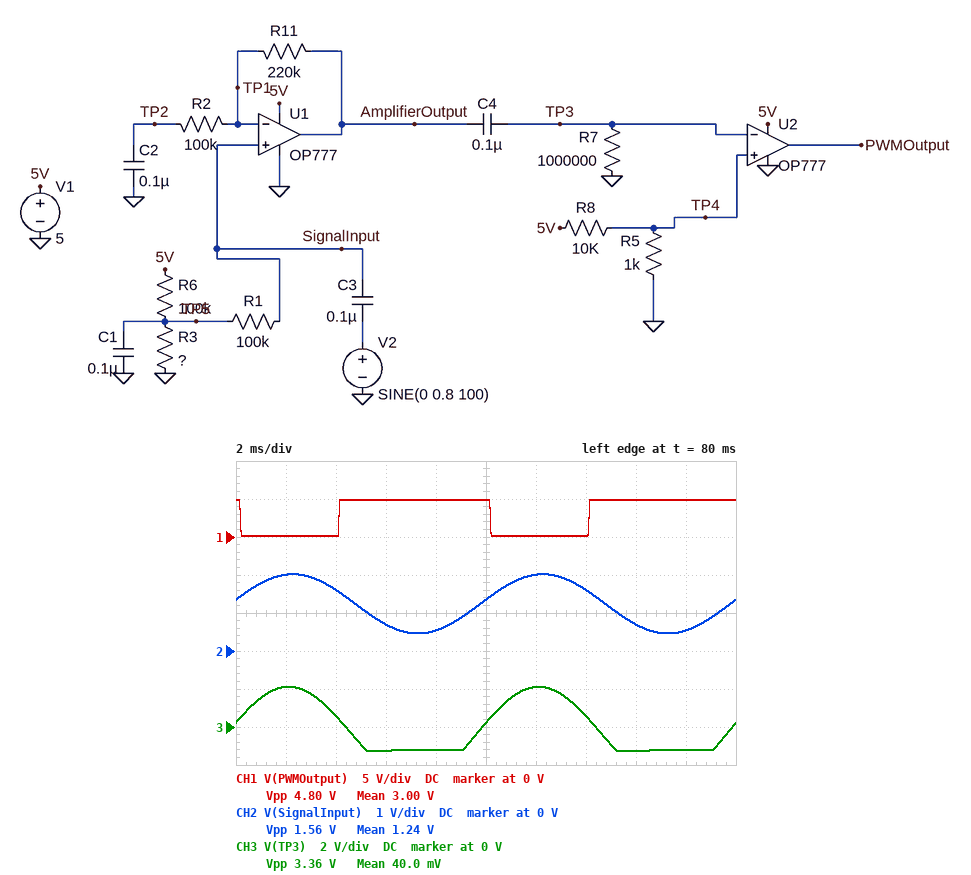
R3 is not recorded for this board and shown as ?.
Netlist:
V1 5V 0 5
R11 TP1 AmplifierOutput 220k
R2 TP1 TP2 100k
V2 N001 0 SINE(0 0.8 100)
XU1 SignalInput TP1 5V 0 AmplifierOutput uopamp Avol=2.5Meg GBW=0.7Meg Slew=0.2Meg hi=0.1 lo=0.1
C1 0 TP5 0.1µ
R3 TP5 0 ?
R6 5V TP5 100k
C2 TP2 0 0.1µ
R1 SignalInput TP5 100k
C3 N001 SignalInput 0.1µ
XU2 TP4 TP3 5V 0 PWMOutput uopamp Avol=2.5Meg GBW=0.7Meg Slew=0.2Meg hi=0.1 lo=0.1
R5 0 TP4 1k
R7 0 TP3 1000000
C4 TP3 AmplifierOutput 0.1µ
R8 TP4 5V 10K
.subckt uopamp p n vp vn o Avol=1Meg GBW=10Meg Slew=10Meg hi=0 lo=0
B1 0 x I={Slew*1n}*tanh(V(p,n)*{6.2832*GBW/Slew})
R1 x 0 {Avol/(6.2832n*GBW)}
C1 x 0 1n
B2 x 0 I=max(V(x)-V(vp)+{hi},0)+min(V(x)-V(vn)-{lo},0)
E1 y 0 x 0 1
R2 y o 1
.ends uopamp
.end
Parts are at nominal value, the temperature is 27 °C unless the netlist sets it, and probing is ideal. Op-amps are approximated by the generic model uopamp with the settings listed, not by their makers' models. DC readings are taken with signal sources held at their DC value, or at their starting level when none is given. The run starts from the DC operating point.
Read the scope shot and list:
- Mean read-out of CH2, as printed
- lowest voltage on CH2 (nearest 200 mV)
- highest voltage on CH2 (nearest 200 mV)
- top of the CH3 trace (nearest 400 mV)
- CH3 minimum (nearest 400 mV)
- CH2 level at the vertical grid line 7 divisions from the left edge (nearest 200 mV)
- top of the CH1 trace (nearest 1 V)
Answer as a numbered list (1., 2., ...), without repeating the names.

1. 1.24 V
2. 400 mV
3. 2.0 V
4. 2.0 V
5. -1.2 V
6. 1.6 V
7. 5 V
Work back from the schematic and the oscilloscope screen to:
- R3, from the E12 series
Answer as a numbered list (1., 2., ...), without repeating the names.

1. 33 kΩ
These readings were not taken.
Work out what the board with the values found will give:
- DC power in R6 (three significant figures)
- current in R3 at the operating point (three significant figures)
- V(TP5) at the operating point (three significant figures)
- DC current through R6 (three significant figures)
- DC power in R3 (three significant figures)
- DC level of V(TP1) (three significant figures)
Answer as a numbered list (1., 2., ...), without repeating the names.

1. 141 µW
2. 37.6 µA
3. 1.24 V
4. 37.6 µA
5. 46.6 µW
6. 1.24 V
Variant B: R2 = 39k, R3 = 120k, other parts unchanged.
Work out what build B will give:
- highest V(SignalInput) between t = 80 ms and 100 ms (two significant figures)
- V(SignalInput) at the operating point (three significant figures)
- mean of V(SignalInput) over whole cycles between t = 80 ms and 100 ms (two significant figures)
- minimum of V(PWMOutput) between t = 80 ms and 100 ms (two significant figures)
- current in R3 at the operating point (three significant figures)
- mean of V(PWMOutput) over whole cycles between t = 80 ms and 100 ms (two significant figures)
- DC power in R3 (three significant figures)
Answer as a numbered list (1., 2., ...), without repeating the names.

1. 3.5 V
2. 2.73 V
3. 2.7 V
4. 100 mV
5. 22.7 µA
6. 2.5 V
7. 62.0 µW
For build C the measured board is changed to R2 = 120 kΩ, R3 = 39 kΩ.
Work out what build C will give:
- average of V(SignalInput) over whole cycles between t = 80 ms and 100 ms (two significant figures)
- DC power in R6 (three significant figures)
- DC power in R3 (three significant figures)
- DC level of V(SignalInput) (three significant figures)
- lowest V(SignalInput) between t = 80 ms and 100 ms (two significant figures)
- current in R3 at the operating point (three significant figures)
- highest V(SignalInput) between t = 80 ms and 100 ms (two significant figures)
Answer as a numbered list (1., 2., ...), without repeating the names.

1. 1.4 V
2. 129 µW
3. 50.5 µW
4. 1.40 V
5. 620 mV
6. 36.0 µA
7. 2.2 V
